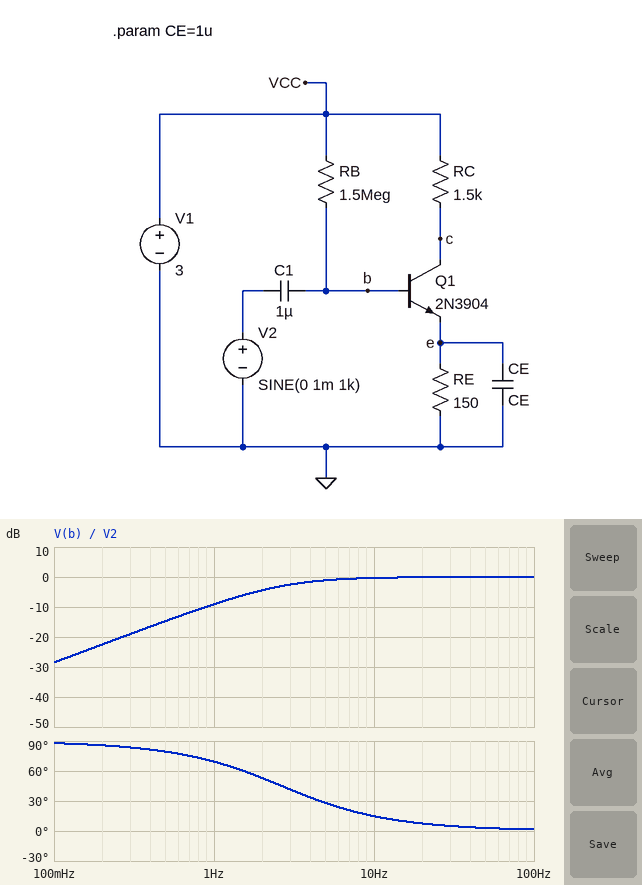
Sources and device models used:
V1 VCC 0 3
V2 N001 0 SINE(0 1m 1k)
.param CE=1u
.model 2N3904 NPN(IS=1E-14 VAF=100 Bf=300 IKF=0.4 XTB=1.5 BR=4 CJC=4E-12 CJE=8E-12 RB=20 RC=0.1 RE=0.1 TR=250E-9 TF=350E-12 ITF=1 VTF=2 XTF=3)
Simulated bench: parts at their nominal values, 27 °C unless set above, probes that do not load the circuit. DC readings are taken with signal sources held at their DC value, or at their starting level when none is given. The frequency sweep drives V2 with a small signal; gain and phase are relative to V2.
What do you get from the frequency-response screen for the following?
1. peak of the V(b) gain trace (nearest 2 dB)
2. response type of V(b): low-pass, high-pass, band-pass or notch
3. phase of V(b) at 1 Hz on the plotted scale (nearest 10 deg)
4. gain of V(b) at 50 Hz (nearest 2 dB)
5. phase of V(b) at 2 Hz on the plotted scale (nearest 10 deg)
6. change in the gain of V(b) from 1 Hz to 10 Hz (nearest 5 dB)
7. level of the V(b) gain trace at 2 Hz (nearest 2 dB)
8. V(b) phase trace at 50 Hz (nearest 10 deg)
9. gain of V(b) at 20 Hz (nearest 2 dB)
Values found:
0 dB
high-pass
70 deg
0 dB
50 deg
10 dB
-4 dB
0 deg
0 dB
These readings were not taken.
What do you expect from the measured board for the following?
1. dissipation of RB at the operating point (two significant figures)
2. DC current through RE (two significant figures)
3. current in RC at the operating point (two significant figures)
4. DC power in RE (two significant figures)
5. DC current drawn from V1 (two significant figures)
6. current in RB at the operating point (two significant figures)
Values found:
3.5 µW
470 µA
470 µA
33 µW
470 µA
1.5 µA
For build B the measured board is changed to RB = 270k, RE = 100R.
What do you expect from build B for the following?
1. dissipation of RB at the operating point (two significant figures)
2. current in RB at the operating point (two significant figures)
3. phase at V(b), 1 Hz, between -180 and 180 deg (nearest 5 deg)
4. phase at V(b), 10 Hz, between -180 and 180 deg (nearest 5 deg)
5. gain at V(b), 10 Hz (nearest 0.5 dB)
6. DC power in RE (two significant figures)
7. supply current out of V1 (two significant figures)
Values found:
17 µW
8.0 µA
90 deg
85 deg
-23.5 dB
320 µW
1.8 mA
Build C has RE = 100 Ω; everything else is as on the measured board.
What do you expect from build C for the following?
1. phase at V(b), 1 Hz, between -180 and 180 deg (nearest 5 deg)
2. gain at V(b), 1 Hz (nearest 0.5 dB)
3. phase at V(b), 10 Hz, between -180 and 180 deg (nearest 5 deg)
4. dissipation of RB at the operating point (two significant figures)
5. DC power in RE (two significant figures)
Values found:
75 deg
-11.0 dB
20 deg
3.6 µW
22 µW
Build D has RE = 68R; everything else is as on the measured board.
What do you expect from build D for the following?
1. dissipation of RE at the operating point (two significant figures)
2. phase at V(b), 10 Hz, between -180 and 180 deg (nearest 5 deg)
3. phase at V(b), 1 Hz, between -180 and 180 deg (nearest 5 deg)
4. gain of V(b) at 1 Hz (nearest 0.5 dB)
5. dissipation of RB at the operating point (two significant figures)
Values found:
15 µW
25 deg
75 deg
-13.0 dB
3.6 µW
